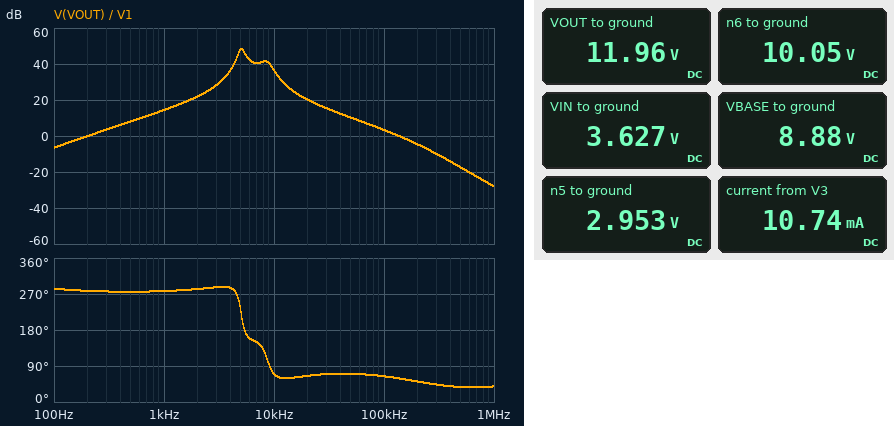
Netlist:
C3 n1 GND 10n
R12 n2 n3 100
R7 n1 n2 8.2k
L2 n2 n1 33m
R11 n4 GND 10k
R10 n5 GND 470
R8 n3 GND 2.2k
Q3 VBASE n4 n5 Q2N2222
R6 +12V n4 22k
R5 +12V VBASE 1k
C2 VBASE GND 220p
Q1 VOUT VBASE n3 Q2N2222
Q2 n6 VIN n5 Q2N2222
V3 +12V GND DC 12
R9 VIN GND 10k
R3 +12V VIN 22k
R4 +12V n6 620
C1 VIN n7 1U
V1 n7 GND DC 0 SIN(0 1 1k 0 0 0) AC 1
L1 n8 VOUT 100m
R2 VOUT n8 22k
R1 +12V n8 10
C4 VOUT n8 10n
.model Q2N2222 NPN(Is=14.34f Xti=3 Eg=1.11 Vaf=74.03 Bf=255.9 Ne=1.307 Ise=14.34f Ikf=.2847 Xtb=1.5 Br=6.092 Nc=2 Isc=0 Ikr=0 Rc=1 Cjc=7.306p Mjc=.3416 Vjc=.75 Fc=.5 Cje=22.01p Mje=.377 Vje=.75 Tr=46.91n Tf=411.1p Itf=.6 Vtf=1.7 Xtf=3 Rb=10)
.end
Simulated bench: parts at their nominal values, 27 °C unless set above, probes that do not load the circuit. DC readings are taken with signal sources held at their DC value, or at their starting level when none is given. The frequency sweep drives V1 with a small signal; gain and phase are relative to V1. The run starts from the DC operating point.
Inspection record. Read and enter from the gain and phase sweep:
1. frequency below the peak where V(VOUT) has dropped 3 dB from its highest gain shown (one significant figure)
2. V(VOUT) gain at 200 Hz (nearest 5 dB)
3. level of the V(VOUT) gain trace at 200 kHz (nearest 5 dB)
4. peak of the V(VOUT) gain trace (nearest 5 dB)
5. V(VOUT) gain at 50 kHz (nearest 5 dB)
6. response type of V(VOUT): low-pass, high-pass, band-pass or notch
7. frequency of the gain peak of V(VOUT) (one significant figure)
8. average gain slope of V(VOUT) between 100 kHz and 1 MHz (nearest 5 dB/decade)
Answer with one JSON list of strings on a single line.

["5 kHz", "0 dB", "-5 dB", "50 dB", "10 dB", "band-pass", "5 kHz", "-30 dB/decade"]
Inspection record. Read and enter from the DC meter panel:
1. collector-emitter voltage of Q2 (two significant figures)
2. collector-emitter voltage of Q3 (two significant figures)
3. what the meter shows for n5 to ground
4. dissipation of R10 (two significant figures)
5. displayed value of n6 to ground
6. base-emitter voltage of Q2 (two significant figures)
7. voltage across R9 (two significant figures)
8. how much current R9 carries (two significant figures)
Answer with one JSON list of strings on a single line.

["7.1 V", "5.9 V", "2.953 V", "19 mW", "10.05 V", "670 mV", "3.6 V", "360 µA"]
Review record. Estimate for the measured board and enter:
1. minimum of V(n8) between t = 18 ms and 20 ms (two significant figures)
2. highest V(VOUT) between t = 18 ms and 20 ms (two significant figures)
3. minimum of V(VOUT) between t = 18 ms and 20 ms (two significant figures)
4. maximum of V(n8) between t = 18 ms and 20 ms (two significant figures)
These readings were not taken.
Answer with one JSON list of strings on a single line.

["12 V", "22 V", "4.3 V", "12 V"]
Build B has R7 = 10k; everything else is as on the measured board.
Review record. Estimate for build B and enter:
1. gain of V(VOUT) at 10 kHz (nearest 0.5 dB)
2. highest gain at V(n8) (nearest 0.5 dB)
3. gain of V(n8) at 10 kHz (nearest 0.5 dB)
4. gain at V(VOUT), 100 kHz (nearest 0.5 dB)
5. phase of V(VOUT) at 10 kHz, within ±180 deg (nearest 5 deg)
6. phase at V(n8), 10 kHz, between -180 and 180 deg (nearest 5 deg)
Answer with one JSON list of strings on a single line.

["37.0 dB", "-6.5 dB", "-9.5 dB", "3.0 dB", "65 deg", "150 deg"]
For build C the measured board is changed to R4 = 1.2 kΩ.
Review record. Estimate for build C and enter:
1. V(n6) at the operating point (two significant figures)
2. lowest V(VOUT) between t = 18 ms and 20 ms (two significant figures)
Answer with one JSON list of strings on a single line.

["8.3 V", "4.4 V"]
